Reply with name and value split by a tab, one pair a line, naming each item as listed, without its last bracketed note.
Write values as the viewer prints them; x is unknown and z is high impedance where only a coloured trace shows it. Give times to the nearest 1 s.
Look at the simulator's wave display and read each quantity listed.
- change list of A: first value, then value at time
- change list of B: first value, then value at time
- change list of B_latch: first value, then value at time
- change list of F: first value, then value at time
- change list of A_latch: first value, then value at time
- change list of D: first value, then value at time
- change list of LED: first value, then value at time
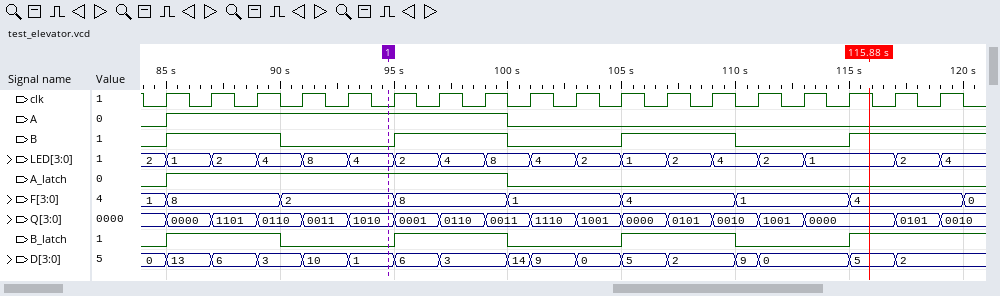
change list of A: first value, then value at time	0, 1 at 85 s, 0 at 100 s
change list of B: first value, then value at time	0, 1 at 85 s, 0 at 90 s, 1 at 95 s, 0 at 100 s, 1 at 105 s, 0 at 110 s, 1 at 115 s
change list of B_latch: first value, then value at time	0, 1 at 85 s, 0 at 90 s, 1 at 95 s, 0 at 100 s, 1 at 105 s, 0 at 110 s, 1 at 115 s
change list of F: first value, then value at time	1, 8 at 85 s, 2 at 90 s, 8 at 95 s, 1 at 100 s, 4 at 105 s, 1 at 110 s, 4 at 115 s, 0 at 120 s
change list of A_latch: first value, then value at time	0, 1 at 85 s, 0 at 100 s
change list of D: first value, then value at time	0, 13 at 85 s, 6 at 87 s, 3 at 89 s, 10 at 91 s, 1 at 93 s, 6 at 95 s, 3 at 97 s, 14 at 100 s, 9 at 101 s, 0 at 103 s, 5 at 105 s, 2 at 107 s, 9 at 110 s, 0 at 111 s, 5 at 115 s, 2 at 117 s
change list of LED: first value, then value at time	2, 1 at 85 s, 2 at 87 s, 4 at 89 s, 8 at 91 s, 4 at 93 s, 2 at 95 s, 4 at 97 s, 8 at 99 s, 4 at 101 s, 2 at 103 s, 1 at 105 s, 2 at 107 s, 4 at 109 s, 2 at 111 s, 1 at 113 s, 2 at 117 s, 4 at 119 s
